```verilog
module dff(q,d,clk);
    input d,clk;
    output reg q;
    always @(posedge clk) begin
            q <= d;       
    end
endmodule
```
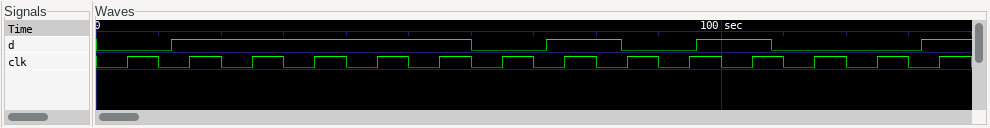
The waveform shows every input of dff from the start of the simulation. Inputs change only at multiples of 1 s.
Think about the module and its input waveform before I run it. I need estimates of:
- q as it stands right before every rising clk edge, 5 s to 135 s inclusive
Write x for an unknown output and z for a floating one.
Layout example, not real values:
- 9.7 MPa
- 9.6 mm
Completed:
- x 0 1 1 1 1 1 0 1 0 0 1 0 0
